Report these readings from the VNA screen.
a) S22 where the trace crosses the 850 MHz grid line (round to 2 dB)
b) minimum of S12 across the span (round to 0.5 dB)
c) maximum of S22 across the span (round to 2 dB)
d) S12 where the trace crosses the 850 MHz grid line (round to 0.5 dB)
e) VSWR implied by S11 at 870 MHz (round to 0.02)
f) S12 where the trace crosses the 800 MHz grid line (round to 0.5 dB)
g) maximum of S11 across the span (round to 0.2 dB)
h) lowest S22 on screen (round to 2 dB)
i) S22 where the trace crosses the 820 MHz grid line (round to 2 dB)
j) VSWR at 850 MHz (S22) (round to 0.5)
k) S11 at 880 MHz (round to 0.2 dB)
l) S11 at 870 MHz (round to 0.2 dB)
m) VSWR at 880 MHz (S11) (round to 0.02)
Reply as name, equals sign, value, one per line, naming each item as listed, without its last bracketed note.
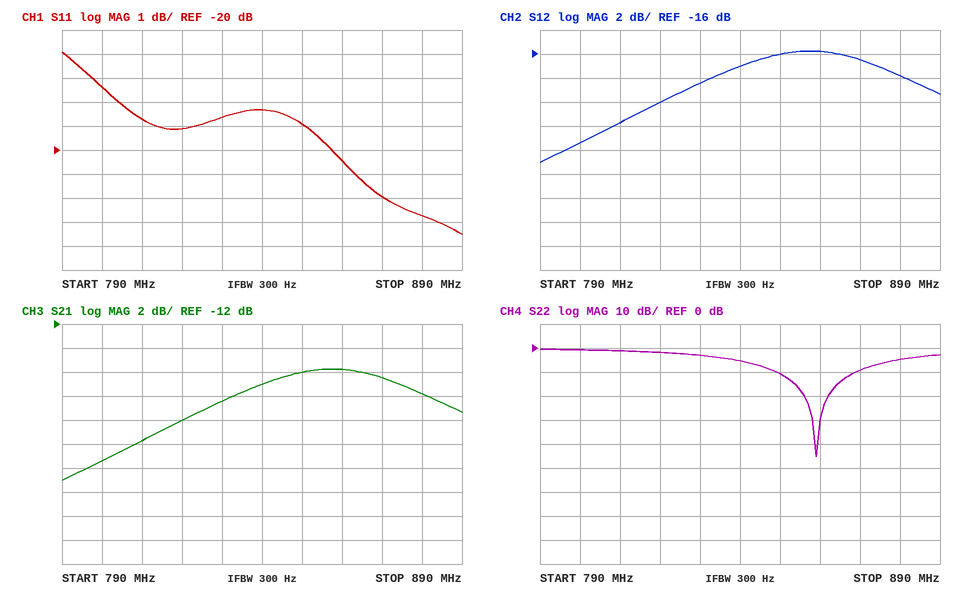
S22 where the trace crosses the 850 MHz grid line = -10 dB
minimum of S12 across the span = -25.0 dB
maximum of S22 across the span = 0 dB
S12 where the trace crosses the 850 MHz grid line = -16.0 dB
VSWR implied by S11 at 870 MHz = 1.18
S12 where the trace crosses the 800 MHz grid line = -23.5 dB
maximum of S11 across the span = -16.0 dB
lowest S22 on screen = -46 dB
S22 where the trace crosses the 820 MHz grid line = -2 dB
VSWR at 850 MHz (S22) = 2.0
S11 at 880 MHz = -22.8 dB
S11 at 870 MHz = -22.0 dB
VSWR at 880 MHz (S11) = 1.16
